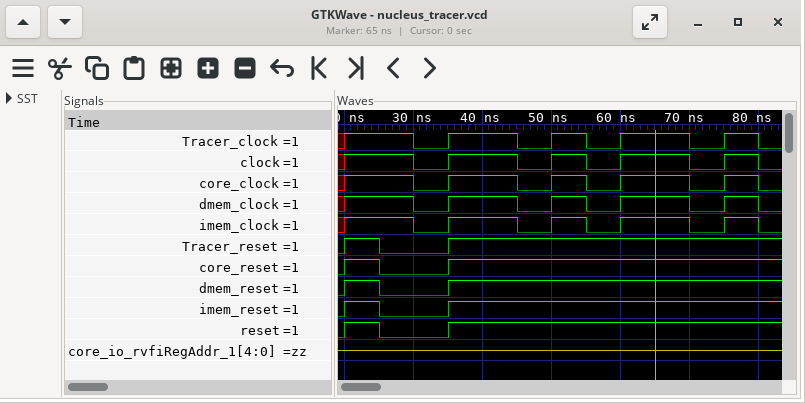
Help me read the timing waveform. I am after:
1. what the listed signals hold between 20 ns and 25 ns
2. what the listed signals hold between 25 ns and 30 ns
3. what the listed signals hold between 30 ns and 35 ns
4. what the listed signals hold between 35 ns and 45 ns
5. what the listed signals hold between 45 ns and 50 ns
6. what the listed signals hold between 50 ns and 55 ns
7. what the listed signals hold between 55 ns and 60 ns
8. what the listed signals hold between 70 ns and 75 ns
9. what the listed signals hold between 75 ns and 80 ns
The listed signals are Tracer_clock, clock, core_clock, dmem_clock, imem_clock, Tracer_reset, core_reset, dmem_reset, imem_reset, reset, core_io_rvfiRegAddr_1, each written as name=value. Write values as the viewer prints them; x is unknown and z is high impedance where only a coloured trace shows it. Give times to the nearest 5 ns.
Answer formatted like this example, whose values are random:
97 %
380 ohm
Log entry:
Tracer_clock=1, clock=1, core_clock=1, dmem_clock=1, imem_clock=1, Tracer_reset=1, core_reset=1, dmem_reset=1, imem_reset=1, reset=1, core_io_rvfiRegAddr_1=z
Tracer_clock=1, clock=1, core_clock=1, dmem_clock=1, imem_clock=1, Tracer_reset=0, core_reset=0, dmem_reset=0, imem_reset=0, reset=0, core_io_rvfiRegAddr_1=z
Tracer_clock=0, clock=0, core_clock=0, dmem_clock=0, imem_clock=0, Tracer_reset=0, core_reset=0, dmem_reset=0, imem_reset=0, reset=0, core_io_rvfiRegAddr_1=z
Tracer_clock=1, clock=1, core_clock=1, dmem_clock=1, imem_clock=1, Tracer_reset=1, core_reset=1, dmem_reset=1, imem_reset=1, reset=1, core_io_rvfiRegAddr_1=z
Tracer_clock=0, clock=0, core_clock=0, dmem_clock=0, imem_clock=0, Tracer_reset=1, core_reset=1, dmem_reset=1, imem_reset=1, reset=1, core_io_rvfiRegAddr_1=z
Tracer_clock=1, clock=1, core_clock=1, dmem_clock=1, imem_clock=1, Tracer_reset=1, core_reset=1, dmem_reset=1, imem_reset=1, reset=1, core_io_rvfiRegAddr_1=z
Tracer_clock=0, clock=0, core_clock=0, dmem_clock=0, imem_clock=0, Tracer_reset=1, core_reset=1, dmem_reset=1, imem_reset=1, reset=1, core_io_rvfiRegAddr_1=z
Tracer_clock=0, clock=0, core_clock=0, dmem_clock=0, imem_clock=0, Tracer_reset=1, core_reset=1, dmem_reset=1, imem_reset=1, reset=1, core_io_rvfiRegAddr_1=z
Tracer_clock=1, clock=1, core_clock=1, dmem_clock=1, imem_clock=1, Tracer_reset=1, core_reset=1, dmem_reset=1, imem_reset=1, reset=1, core_io_rvfiRegAddr_1=z
